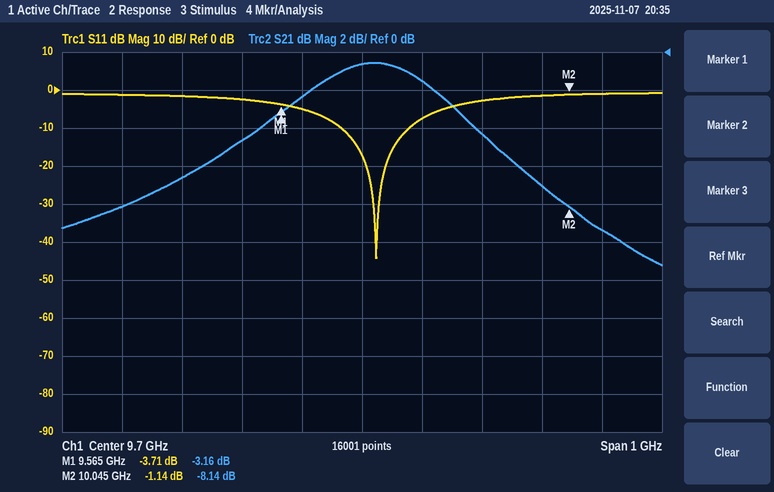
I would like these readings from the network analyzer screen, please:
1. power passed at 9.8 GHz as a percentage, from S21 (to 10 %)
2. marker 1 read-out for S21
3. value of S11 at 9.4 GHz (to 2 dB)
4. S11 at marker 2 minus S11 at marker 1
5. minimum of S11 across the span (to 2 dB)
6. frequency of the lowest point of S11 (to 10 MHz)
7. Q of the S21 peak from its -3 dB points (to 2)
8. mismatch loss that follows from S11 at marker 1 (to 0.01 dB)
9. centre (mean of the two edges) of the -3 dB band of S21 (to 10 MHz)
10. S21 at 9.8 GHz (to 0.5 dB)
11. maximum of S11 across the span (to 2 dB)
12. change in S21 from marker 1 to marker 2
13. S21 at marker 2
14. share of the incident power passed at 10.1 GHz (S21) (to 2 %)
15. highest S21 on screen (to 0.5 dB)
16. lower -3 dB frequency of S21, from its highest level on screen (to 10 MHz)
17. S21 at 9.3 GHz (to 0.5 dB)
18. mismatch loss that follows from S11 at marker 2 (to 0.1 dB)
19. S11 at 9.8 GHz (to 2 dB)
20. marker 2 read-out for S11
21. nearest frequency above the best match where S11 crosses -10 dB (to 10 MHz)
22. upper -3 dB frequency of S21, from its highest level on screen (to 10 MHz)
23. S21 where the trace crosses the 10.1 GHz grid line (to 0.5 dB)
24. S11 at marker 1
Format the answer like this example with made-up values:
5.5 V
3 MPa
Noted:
70 %
-3.16 dB
-2 dB
2.57 dB
-44 dB
9.72 GHz
30
2.41 dB
9.71 GHz
-1.5 dB
0 dB
-4.98 dB
-8.14 dB
12 %
-0.5 dB
9.55 GHz
-8.0 dB
6.4 dB
-8 dB
-1.14 dB
9.78 GHz
9.87 GHz
-9.5 dB
-3.71 dB
